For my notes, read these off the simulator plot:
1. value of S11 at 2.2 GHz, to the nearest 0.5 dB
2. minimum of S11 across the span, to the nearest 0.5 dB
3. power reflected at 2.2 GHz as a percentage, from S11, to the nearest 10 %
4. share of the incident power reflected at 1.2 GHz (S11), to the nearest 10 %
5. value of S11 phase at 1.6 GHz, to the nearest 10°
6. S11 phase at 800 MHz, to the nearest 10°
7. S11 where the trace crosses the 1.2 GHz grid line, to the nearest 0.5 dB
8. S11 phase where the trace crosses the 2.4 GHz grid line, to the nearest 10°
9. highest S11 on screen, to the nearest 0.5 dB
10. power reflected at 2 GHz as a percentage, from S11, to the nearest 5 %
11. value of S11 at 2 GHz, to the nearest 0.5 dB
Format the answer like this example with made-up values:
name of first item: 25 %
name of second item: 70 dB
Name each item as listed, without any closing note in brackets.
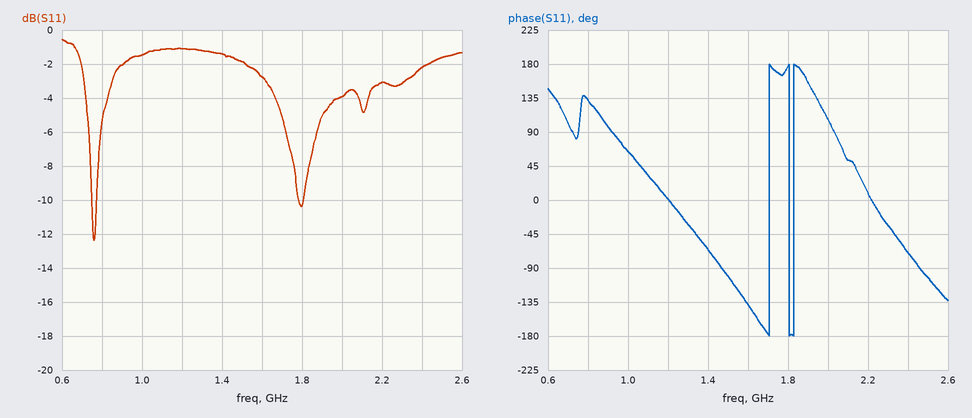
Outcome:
value of S11 at 2.2 GHz, to the nearest 0.5 dB: -3.0 dB
minimum of S11 across the span, to the nearest 0.5 dB: -12.5 dB
power reflected at 2.2 GHz as a percentage, from S11, to the nearest 10 %: 50 %
share of the incident power reflected at 1.2 GHz (S11), to the nearest 10 %: 80 %
value of S11 phase at 1.6 GHz, to the nearest 10°: -140°
S11 phase at 800 MHz, to the nearest 10°: 130°
S11 where the trace crosses the 1.2 GHz grid line, to the nearest 0.5 dB: -1.0 dB
S11 phase where the trace crosses the 2.4 GHz grid line, to the nearest 10°: -70°
highest S11 on screen, to the nearest 0.5 dB: -0.5 dB
power reflected at 2 GHz as a percentage, from S11, to the nearest 5 %: 40 %
value of S11 at 2 GHz, to the nearest 0.5 dB: -4.0 dB
